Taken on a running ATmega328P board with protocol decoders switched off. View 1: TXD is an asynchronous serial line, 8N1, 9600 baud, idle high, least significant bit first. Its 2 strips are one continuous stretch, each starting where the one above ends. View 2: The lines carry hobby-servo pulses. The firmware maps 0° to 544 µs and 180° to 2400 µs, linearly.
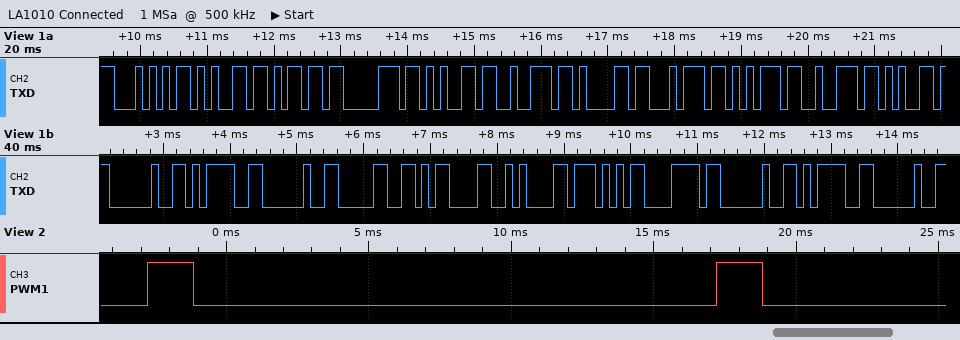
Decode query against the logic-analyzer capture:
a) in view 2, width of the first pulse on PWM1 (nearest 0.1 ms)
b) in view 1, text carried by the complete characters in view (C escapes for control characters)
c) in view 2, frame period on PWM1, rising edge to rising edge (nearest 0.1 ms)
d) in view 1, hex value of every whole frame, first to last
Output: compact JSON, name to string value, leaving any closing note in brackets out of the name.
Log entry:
{"in view 2, width of the first pulse on PWM1": "1.6 ms", "in view 1, text carried by the complete characters in view": "\"Temperature = 0\\r\\nWx = \"", "in view 2, frame period on PWM1, rising edge to rising edge": "20.0 ms", "in view 1, hex value of every whole frame, first to last": "54 65 6D 70 65 72 61 74 75 72 65 20 3D 20 30 0D 0A 57 78 20 3D 20"}
